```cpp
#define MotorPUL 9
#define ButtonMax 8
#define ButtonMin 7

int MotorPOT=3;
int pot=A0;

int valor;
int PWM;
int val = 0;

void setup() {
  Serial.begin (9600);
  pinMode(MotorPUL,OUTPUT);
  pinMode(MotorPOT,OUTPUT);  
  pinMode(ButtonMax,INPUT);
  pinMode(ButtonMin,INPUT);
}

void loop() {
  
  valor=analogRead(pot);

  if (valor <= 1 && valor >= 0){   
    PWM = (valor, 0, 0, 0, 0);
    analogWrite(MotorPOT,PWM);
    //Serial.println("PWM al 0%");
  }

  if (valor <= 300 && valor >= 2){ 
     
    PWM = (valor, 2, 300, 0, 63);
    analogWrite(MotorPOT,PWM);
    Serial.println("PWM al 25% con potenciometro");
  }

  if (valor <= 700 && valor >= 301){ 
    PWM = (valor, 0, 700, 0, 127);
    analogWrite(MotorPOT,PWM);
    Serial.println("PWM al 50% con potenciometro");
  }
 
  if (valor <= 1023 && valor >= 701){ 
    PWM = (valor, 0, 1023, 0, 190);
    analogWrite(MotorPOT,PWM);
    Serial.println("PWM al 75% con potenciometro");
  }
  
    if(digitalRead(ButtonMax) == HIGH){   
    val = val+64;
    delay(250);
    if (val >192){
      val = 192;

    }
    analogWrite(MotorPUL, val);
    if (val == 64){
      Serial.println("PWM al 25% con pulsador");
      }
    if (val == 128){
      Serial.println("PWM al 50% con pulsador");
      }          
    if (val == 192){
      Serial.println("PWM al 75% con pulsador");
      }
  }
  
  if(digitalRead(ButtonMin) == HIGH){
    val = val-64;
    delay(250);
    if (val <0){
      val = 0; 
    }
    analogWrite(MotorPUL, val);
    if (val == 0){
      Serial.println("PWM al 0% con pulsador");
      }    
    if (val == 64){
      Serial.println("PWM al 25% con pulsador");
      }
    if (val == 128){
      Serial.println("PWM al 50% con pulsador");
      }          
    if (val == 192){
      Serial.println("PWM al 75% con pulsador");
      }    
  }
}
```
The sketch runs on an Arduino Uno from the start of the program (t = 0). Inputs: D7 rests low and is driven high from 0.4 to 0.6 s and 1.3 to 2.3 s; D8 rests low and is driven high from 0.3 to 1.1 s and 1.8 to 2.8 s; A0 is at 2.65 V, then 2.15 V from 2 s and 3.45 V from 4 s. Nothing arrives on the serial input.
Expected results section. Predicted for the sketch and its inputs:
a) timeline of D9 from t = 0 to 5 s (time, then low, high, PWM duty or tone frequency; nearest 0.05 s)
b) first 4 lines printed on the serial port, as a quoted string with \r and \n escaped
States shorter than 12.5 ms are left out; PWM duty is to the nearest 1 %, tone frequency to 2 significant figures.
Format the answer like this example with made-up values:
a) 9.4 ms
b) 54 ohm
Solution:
a) 0 s low; 0.55 s PWM 25 %; 0.8 s low; 1.05 s PWM 25 %; 1.3 s PWM 50 %; 1.55 s PWM 25 %; 1.8 s low; 2.05 s PWM 25 %; 2.3 s low; 2.55 s PWM 25 %; 2.8 s PWM 50 %
b) "PWM al 50% con potenciometro\r\nPWM al 50% con potenciometro\r\nPWM al 50% con potenciometro\r\nPWM al 50% con potenciometro\r\n"
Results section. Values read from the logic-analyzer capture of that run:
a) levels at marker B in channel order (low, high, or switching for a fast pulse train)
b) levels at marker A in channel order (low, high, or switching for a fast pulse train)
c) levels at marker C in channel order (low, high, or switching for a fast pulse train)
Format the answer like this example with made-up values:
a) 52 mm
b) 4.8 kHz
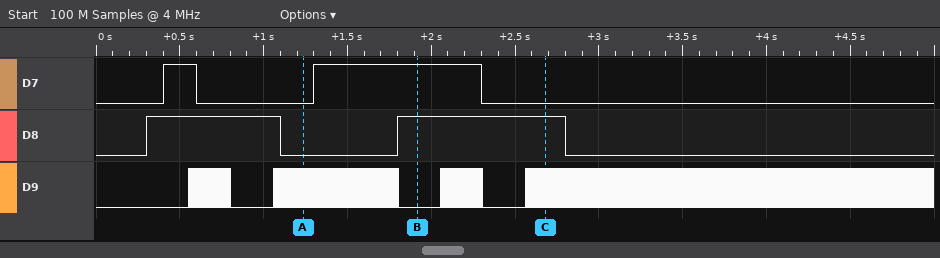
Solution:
a) D7 high, D8 high, D9 low
b) D7 low, D8 low, D9 switching
c) D7 low, D8 high, D9 switching
